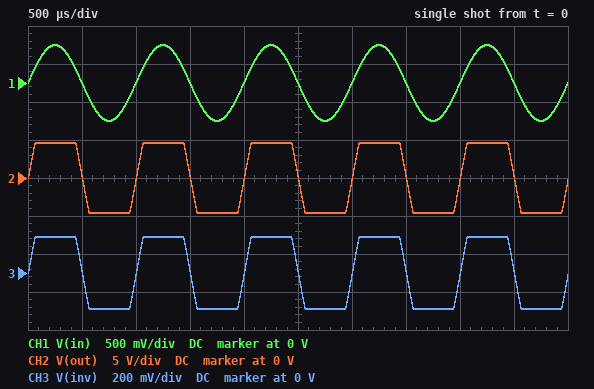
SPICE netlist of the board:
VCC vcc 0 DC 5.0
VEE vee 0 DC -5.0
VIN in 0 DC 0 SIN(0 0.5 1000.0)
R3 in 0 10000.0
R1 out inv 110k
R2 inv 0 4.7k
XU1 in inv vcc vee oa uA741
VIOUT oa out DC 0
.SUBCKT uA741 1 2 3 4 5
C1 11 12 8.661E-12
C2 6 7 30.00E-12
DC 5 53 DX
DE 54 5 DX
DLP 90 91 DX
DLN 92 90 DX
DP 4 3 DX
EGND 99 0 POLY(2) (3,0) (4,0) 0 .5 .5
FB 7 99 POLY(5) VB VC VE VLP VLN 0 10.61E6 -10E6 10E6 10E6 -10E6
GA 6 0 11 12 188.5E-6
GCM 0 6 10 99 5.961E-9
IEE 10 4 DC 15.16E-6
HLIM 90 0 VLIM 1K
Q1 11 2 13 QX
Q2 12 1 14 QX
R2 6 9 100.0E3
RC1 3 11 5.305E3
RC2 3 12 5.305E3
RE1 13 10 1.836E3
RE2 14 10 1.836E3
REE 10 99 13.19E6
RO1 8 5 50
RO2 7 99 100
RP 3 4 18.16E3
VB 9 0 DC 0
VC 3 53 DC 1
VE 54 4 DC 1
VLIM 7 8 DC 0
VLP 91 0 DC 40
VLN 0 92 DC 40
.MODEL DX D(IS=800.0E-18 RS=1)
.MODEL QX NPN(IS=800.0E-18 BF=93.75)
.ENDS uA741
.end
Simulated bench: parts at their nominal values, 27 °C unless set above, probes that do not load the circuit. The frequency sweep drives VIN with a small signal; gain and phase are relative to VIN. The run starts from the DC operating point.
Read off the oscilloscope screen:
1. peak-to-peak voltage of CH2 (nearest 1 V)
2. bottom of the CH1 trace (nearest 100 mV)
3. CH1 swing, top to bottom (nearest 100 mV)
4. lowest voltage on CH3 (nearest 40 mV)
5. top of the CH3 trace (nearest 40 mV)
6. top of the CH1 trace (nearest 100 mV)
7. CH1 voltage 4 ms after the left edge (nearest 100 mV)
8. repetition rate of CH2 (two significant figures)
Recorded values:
9 V
-500 mV
1.0 V
-200 mV
200 mV
500 mV
0 V
1.0 kHz
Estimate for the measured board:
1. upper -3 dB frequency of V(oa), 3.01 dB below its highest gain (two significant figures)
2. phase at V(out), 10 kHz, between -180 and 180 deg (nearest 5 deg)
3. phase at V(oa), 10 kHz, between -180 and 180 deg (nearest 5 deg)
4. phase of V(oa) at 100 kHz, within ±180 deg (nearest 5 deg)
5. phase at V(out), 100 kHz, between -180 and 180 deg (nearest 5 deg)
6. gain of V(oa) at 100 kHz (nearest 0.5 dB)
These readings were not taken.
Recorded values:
42 kHz
-15 deg
-15 deg
-70 deg
-70 deg
19.5 dB
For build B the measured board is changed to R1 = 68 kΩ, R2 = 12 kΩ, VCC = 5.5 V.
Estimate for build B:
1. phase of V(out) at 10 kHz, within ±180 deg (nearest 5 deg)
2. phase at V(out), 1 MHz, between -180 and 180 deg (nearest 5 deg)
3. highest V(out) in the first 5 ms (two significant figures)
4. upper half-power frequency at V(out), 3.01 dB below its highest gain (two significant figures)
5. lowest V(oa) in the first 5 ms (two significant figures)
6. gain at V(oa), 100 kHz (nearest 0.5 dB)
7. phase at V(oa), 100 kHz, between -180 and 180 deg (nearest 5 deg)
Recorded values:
-5 deg
-115 deg
3.3 V
160 kHz
-3.3 V
15.0 dB
-35 deg
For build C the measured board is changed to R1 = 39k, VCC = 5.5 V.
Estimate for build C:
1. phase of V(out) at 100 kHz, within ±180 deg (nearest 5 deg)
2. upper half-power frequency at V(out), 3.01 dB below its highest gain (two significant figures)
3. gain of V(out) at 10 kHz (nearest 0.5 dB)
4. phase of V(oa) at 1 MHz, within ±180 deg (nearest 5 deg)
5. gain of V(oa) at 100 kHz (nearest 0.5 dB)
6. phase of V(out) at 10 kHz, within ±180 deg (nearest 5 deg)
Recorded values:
-45 deg
110 kHz
19.5 dB
-115 deg
17.0 dB
-5 deg
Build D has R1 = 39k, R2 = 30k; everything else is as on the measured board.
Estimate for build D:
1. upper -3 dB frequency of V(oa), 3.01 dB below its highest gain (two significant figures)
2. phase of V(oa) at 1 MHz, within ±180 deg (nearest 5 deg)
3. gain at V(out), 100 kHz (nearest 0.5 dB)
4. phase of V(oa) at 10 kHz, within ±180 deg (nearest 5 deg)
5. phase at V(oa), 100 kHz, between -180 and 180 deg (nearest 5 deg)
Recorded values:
550 kHz
-100 deg
7.0 dB
0 deg
-15 deg
